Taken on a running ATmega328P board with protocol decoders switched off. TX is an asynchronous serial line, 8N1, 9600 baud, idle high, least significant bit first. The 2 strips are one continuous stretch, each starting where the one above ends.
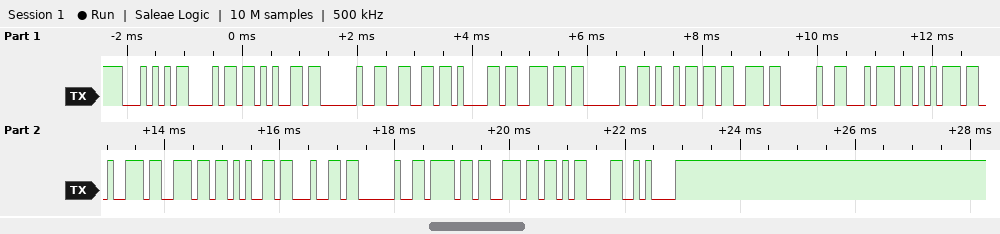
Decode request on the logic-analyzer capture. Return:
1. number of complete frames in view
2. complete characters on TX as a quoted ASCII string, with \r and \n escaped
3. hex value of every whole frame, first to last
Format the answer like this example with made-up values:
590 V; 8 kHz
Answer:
22; "The fan is turned on\r\n"; 0x54 0x68 0x65 0x20 0x66 0x61 0x6E 0x20 0x69 0x73 0x20 0x74 0x75 0x72 0x6E 0x65 0x64 0x20 0x6F 0x6E 0x0D 0x0A
